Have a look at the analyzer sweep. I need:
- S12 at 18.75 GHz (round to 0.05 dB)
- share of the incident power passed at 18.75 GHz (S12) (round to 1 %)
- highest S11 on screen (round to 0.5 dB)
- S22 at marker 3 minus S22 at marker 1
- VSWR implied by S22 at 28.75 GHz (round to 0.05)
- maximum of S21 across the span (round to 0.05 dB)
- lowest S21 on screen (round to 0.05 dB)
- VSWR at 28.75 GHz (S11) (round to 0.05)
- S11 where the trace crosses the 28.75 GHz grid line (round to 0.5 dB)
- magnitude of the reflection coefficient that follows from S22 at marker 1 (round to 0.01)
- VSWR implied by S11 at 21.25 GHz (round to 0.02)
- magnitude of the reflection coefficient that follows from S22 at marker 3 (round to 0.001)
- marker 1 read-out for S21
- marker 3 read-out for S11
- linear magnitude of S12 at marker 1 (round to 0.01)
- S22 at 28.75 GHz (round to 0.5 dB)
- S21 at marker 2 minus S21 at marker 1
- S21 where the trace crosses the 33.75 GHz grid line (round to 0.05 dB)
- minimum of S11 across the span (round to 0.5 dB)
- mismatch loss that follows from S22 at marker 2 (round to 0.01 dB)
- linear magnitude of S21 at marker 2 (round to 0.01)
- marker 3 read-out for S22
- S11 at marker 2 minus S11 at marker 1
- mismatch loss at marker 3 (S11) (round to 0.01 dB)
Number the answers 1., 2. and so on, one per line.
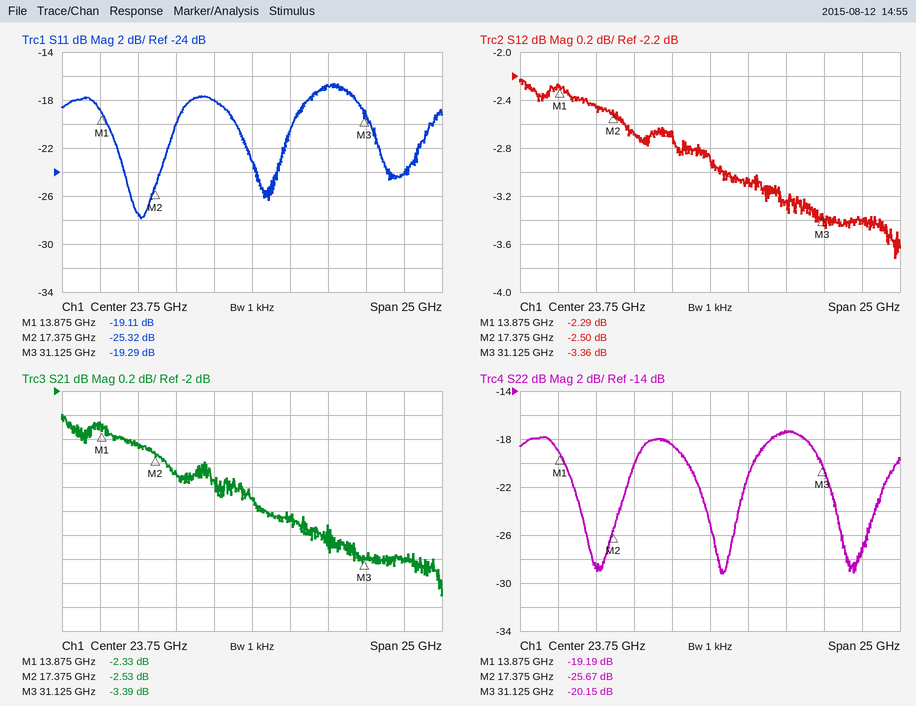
1. -2.70 dB
2. 54 %
3. -16.5 dB
4. -0.96 dB
5. 1.30
6. -2.20 dB
7. -3.70 dB
8. 1.35
9. -17.0 dB
10. 0.11
11. 1.28
12. 0.098
13. -2.33 dB
14. -19.29 dB
15. 0.77
16. -17.5 dB
17. -0.20 dB
18. -3.40 dB
19. -28.0 dB
20. 0.01 dB
21. 0.75
22. -20.15 dB
23. -6.21 dB
24. 0.05 dB
